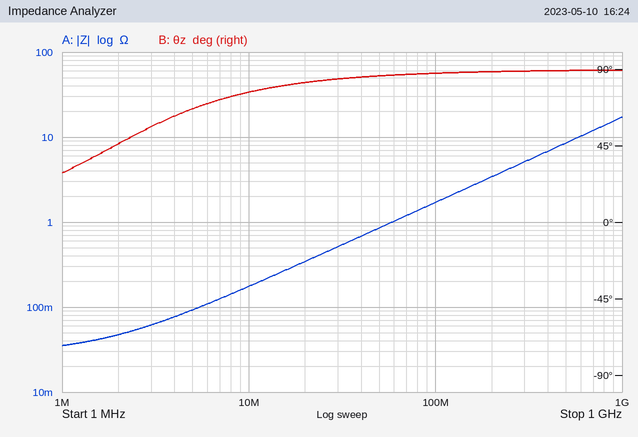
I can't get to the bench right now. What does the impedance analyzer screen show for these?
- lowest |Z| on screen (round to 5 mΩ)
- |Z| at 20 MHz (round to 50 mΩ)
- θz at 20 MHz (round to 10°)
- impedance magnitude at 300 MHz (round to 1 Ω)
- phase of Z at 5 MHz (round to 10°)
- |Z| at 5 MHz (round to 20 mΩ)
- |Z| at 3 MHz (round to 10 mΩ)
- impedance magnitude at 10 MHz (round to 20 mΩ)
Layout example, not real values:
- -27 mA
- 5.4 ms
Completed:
- 35 mΩ
- 350 mΩ
- 80°
- 5 Ω
- 70°
- 100 mΩ
- 60 mΩ
- 180 mΩ
